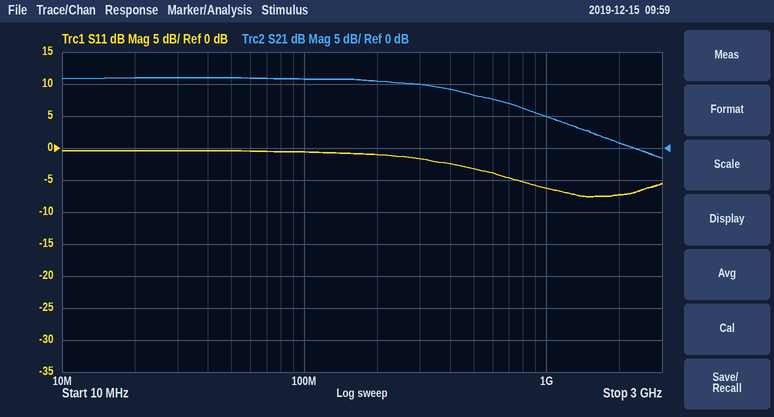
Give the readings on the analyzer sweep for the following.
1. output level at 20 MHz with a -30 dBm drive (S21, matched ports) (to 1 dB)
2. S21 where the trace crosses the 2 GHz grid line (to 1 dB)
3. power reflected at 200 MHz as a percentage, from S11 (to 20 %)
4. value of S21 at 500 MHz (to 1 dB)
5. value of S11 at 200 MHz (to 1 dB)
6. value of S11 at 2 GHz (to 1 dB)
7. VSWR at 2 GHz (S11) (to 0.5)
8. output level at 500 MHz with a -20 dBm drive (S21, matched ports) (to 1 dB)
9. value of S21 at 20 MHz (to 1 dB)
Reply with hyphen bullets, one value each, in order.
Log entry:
- -19 dBm
- 1 dB
- 80 %
- 8 dB
- -1 dB
- -7 dB
- 2.5
- -12 dBm
- 11 dB
